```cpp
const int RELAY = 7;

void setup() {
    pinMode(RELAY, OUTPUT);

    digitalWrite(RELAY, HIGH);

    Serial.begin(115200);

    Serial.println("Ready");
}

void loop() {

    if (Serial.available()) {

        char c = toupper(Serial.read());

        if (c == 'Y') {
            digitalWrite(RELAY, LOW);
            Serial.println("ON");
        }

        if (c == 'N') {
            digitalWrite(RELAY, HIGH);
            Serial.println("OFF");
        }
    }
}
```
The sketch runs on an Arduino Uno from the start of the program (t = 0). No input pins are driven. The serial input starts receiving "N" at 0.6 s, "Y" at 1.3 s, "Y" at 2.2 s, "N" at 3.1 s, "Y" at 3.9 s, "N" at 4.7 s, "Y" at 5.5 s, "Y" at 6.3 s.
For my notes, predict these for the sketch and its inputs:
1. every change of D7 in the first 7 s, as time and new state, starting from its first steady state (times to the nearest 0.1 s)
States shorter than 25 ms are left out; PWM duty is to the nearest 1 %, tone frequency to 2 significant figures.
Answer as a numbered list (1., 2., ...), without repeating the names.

1. 0 s high; 1.3 s low; 3.1 s high; 3.9 s low; 4.7 s high; 5.5 s low
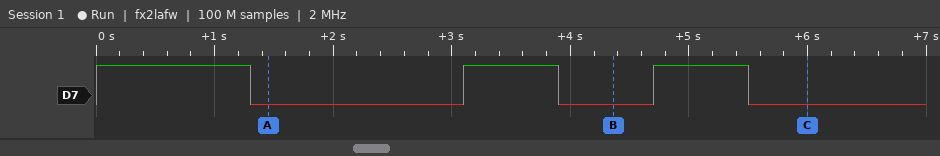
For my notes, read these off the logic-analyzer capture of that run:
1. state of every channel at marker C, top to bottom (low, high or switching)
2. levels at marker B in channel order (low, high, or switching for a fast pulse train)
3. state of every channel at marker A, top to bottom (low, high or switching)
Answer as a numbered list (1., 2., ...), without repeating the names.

1. D7 low
2. D7 low
3. D7 low
